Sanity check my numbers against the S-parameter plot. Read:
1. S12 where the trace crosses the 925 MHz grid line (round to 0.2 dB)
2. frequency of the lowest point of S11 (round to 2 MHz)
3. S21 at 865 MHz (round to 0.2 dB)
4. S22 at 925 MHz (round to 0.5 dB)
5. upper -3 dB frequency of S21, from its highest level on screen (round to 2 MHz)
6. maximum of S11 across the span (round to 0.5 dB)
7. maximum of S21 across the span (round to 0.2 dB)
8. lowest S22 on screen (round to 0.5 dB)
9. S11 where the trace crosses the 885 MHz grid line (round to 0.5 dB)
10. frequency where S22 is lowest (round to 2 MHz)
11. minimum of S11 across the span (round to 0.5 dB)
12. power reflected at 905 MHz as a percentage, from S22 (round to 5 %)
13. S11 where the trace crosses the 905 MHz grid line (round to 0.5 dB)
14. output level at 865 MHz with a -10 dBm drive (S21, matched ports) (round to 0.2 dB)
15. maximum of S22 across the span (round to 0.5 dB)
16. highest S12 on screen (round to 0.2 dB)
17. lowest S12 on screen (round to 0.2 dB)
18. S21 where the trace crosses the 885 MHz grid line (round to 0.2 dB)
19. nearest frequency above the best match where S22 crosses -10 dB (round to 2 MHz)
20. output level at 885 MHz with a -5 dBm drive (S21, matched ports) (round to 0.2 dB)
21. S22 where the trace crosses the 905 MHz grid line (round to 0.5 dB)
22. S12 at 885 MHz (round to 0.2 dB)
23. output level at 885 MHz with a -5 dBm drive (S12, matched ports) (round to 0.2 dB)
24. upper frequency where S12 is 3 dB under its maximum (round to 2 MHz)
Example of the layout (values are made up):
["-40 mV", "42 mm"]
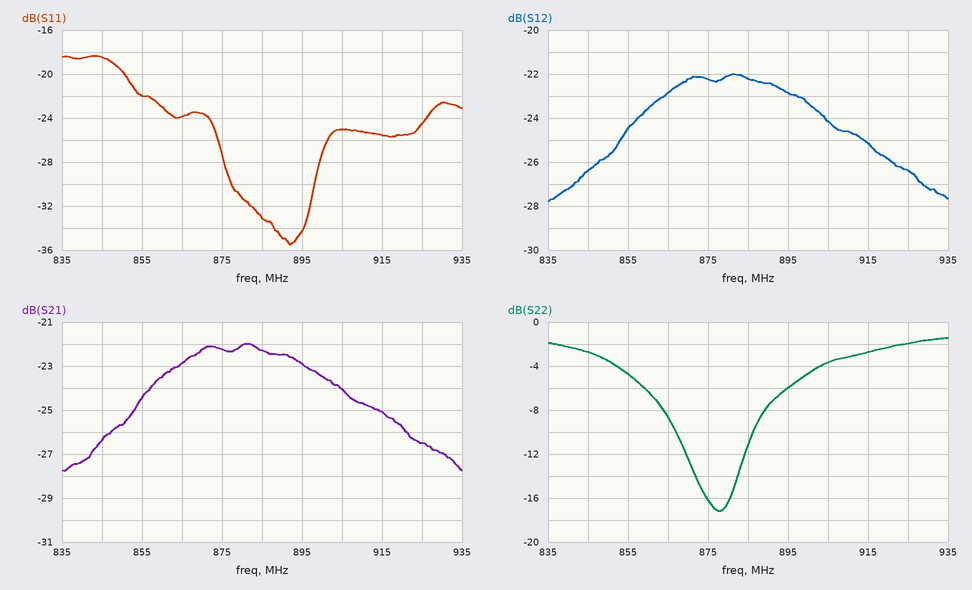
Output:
["-26.4 dB", "892 MHz", "-22.8 dB", "-2.0 dB", "914 MHz", "-18.5 dB", "-22.0 dB", "-17.0 dB", "-33.0 dB", "878 MHz", "-35.5 dB", "45 %", "-25.0 dB", "-32.8 dBm", "-1.5 dB", "-22.0 dB", "-27.8 dB", "-22.2 dB", "886 MHz", "-27.2 dBm", "-3.5 dB", "-22.2 dB", "-27.2 dBm", "914 MHz"]
